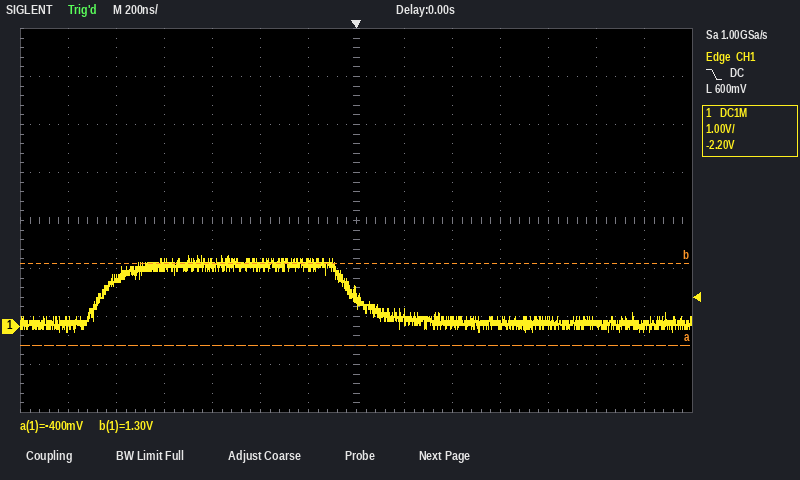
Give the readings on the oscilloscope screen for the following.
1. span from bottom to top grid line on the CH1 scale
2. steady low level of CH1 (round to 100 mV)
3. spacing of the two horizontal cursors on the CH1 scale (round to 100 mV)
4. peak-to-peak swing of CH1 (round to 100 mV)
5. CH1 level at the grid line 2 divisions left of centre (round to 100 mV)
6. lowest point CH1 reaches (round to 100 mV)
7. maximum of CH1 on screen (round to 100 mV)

8 V
100 mV
1.7 V
1.6 V
1.2 V
-100 mV
1.5 V
